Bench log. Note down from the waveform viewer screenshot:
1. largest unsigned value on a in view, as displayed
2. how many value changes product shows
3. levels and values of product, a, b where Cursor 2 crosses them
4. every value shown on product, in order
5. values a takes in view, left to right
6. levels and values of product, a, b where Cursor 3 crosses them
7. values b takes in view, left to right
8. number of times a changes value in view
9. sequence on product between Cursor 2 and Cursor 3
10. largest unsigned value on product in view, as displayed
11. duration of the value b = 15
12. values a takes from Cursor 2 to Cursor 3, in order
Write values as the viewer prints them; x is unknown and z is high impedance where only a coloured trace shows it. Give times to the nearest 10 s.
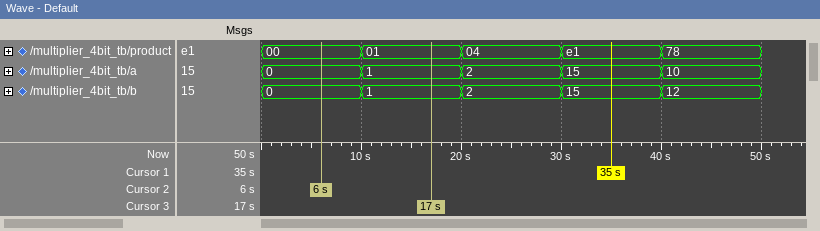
15
4
product=00, a=0, b=0
00, 01, 04, e1, 78
0, 1, 2, 15, 10
product=01, a=1, b=1
0, 1, 2, 15, 12
4
00, 01
e1
10 s
0, 1
